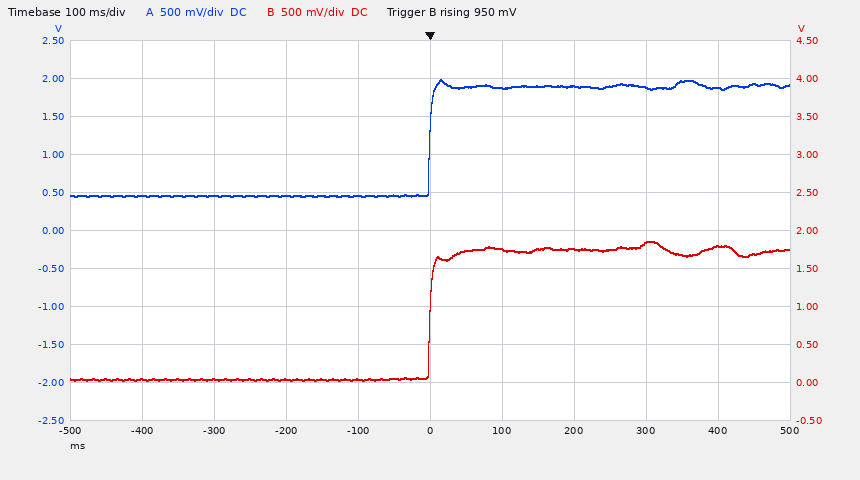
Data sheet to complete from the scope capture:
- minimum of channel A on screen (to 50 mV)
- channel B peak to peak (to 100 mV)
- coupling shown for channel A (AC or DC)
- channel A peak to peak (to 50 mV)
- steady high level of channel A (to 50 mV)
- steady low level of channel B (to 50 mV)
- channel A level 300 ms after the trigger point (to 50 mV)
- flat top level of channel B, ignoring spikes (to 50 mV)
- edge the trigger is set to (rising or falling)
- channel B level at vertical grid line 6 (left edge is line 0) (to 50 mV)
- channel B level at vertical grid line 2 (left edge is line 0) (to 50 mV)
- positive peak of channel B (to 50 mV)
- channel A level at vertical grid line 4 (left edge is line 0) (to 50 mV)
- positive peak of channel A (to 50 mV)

450 mV
1.80 V
DC
1.55 V
1.90 V
50 mV
1.90 V
1.75 V
rising
1.75 V
50 mV
1.85 V
450 mV
2.00 V
